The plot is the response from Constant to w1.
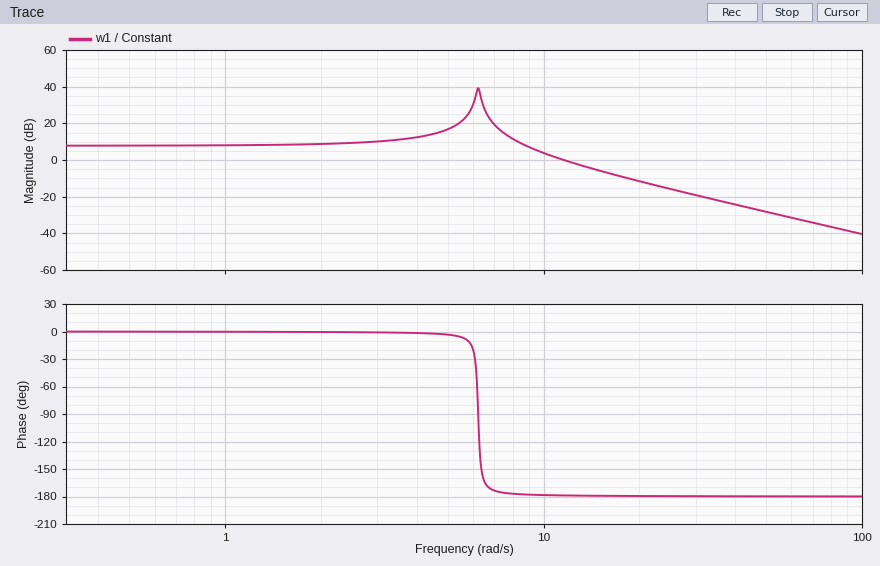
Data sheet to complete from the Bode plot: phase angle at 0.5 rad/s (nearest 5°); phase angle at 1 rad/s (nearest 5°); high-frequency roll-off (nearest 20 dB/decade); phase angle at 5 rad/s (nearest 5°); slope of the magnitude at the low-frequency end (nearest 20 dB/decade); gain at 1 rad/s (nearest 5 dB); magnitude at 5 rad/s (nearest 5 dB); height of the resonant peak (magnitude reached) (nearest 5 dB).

0°
0°
-40 dB/decade
-5°
0 dB/decade
10 dB
15 dB
40 dB
